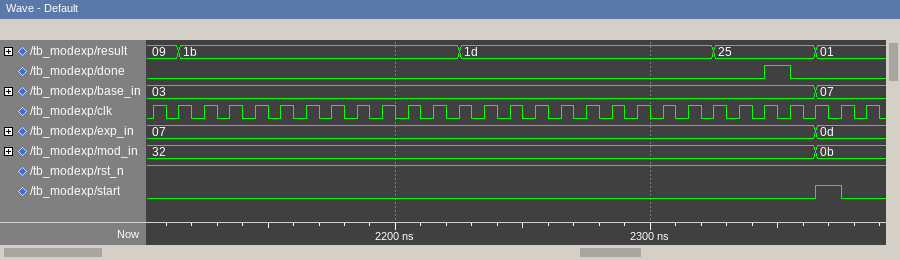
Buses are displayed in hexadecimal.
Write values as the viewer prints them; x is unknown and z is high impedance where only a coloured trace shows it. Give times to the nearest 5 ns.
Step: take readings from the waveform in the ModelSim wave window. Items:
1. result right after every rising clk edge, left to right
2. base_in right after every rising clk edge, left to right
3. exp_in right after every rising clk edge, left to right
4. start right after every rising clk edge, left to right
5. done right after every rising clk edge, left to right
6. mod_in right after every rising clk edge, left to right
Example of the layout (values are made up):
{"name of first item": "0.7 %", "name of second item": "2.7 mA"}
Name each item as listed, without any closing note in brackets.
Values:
{"result right after every rising clk edge, left to right": "09, 1b, 1b, 1b, 1b, 1b, 1b, 1b, 1b, 1b, 1b, 1b, 1d, 1d, 1d, 1d, 1d, 1d, 1d, 1d, 1d, 1d, 25, 25, 25, 25, 01, 01, 01", "base_in right after every rising clk edge, left to right": "03, 03, 03, 03, 03, 03, 03, 03, 03, 03, 03, 03, 03, 03, 03, 03, 03, 03, 03, 03, 03, 03, 03, 03, 03, 03, 07, 07, 07", "exp_in right after every rising clk edge, left to right": "07, 07, 07, 07, 07, 07, 07, 07, 07, 07, 07, 07, 07, 07, 07, 07, 07, 07, 07, 07, 07, 07, 07, 07, 07, 07, 0d, 0d, 0d", "start right after every rising clk edge, left to right": "0 0 0 0 0 0 0 0 0 0 0 0 0 0 0 0 0 0 0 0 0 0 0 0 0 0 1 0 0", "done right after every rising clk edge, left to right": "0 0 0 0 0 0 0 0 0 0 0 0 0 0 0 0 0 0 0 0 0 0 0 0 1 0 0 0 0", "mod_in right after every rising clk edge, left to right": "32, 32, 32, 32, 32, 32, 32, 32, 32, 32, 32, 32, 32, 32, 32, 32, 32, 32, 32, 32, 32, 32, 32, 32, 32, 32, 0b, 0b, 0b"}
